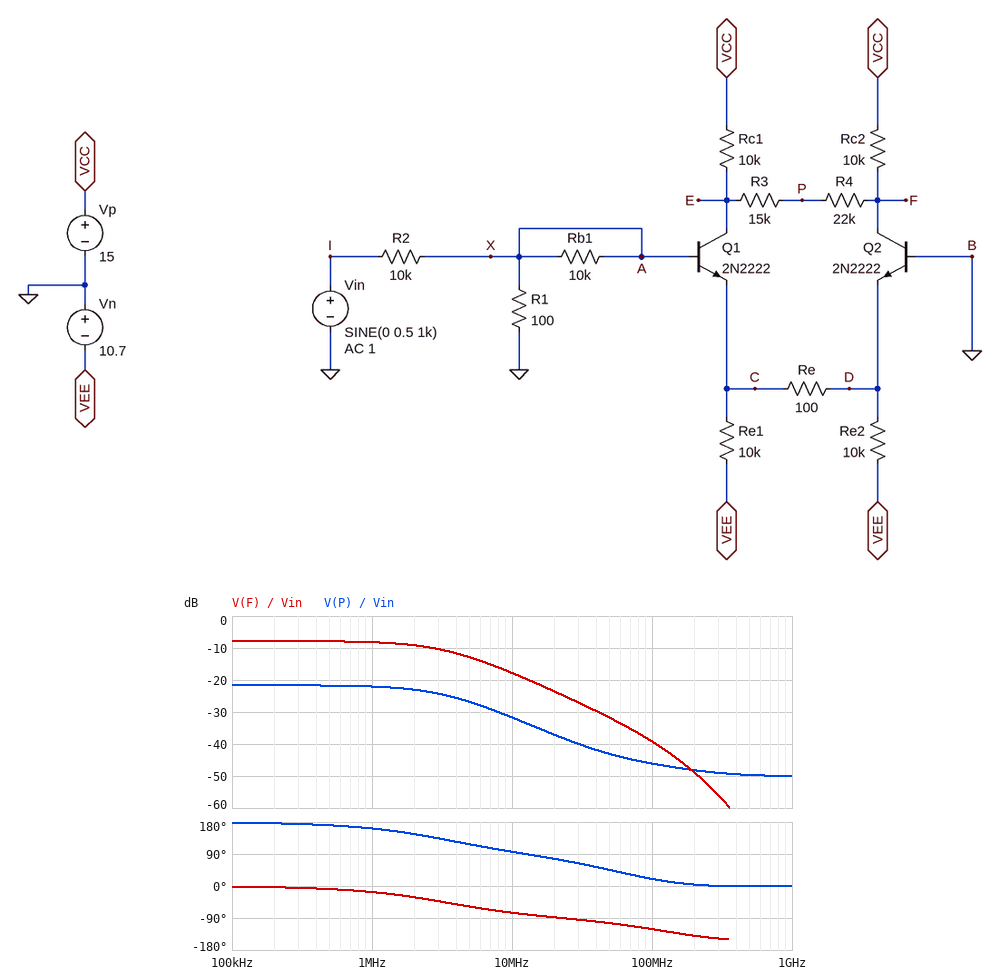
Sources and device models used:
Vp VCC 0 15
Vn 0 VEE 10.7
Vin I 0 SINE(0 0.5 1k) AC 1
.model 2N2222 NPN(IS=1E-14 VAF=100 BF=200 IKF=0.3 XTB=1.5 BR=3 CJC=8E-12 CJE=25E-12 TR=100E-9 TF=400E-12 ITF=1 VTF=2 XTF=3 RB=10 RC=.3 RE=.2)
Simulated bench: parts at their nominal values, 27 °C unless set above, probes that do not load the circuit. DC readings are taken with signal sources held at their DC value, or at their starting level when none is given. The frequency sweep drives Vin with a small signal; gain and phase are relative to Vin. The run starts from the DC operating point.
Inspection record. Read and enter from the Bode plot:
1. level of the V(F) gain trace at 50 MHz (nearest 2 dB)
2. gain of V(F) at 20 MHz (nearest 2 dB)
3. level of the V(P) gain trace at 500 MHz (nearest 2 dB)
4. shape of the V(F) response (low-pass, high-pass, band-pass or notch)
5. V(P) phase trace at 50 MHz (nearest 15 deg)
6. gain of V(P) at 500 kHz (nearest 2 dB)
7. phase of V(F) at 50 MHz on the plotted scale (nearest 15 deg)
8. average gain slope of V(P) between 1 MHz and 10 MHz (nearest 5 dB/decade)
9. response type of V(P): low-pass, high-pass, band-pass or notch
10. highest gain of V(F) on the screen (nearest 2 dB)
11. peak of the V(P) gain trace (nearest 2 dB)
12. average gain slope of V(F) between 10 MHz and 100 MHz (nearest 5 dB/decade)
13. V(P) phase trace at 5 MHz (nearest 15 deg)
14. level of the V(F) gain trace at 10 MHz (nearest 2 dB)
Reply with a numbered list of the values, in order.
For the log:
1. -32 dB
2. -24 dB
3. -50 dB
4. low-pass
5. 45 deg
6. -22 dB
7. -105 deg
8. -10 dB/decade
9. low-pass
10. -8 dB
11. -22 dB
12. -20 dB/decade
13. 120 deg
14. -18 dB
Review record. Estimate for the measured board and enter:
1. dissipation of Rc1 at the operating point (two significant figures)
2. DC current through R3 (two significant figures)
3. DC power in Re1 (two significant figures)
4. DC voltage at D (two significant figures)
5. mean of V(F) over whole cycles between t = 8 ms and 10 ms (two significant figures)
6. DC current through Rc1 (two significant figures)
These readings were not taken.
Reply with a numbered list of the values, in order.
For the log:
1. 10 mW
2. 1.1 µA
3. 10 mW
4. -650 mV
5. 5.0 V
6. 1.0 mA
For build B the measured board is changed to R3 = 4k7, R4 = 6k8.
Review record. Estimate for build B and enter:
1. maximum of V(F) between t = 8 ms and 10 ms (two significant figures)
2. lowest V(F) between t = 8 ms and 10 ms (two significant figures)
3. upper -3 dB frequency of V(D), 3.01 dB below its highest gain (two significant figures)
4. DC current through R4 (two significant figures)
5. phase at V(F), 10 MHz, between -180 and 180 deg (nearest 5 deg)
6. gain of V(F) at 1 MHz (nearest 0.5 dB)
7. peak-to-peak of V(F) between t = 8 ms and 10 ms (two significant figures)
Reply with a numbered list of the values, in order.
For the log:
1. 5.1 V
2. 4.9 V
3. 45 MHz
4. 1.9 µA
5. -65 deg
6. -13.0 dB
7. 230 mV
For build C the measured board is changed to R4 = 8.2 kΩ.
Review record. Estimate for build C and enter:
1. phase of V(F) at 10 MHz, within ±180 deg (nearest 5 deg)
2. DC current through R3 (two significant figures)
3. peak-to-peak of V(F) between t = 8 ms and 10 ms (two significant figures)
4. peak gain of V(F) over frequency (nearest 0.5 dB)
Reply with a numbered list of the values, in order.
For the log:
1. -70 deg
2. 1.4 µA
3. 340 mV
4. -9.5 dB
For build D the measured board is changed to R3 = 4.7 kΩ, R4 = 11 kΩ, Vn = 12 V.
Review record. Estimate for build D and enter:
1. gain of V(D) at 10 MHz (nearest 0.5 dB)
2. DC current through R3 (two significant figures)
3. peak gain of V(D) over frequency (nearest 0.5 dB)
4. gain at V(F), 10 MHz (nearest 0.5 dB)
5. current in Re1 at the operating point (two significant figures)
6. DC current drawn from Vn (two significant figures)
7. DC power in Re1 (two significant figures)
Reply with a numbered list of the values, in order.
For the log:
1. -58.0 dB
2. 2.0 µA
3. -56.0 dB
4. -18.5 dB
5. 1.1 mA
6. 2.3 mA
7. 13 mW
